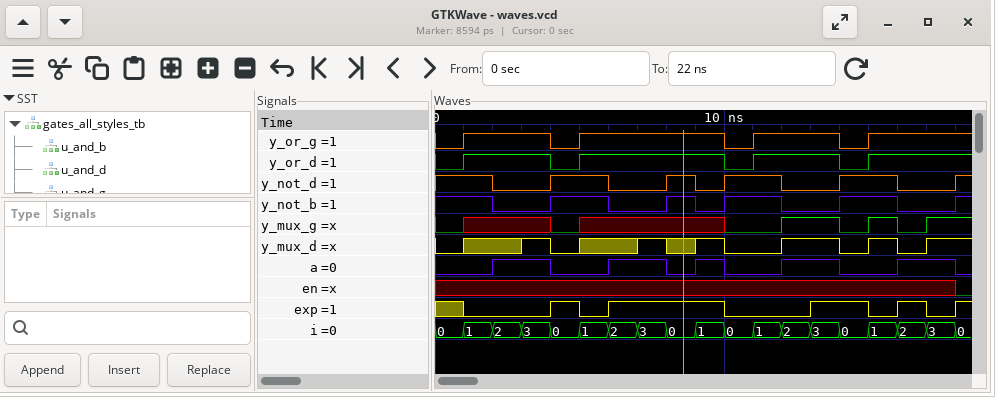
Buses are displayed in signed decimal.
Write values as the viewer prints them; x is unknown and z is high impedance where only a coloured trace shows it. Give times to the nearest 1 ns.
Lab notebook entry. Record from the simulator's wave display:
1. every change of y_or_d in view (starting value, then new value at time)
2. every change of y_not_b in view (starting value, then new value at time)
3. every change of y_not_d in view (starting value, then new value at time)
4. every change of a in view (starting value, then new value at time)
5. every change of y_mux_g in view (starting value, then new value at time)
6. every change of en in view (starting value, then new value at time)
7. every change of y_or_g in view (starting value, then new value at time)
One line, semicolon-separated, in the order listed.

0, 1 at 1 ns, 0 at 4 ns, 1 at 5 ns, 0 at 10 ns, 1 at 11 ns, 0 at 14 ns, 1 at 15 ns; 1, 0 at 2 ns, 1 at 4 ns, 0 at 6 ns, 1 at 8 ns, 0 at 9 ns, 1 at 10 ns, 0 at 12 ns, 1 at 14 ns, 0 at 16 ns, 1 at 18 ns; 1, 0 at 2 ns, 1 at 4 ns, 0 at 6 ns, 1 at 8 ns, 0 at 9 ns, 1 at 10 ns, 0 at 12 ns, 1 at 14 ns, 0 at 16 ns, 1 at 18 ns; 0, 1 at 2 ns, 0 at 4 ns, 1 at 6 ns, 0 at 8 ns, 1 at 9 ns, 0 at 10 ns, 1 at 12 ns, 0 at 14 ns, 1 at 16 ns, 0 at 18 ns; 0, x at 1 ns, 0 at 4 ns, x at 5 ns, 0 at 10 ns, 1 at 12 ns, 0 at 14 ns, 1 at 15 ns, 0 at 16 ns, 1 at 17 ns; x, 0 at 18 ns; 0, 1 at 1 ns, 0 at 4 ns, 1 at 5 ns, 0 at 10 ns, 1 at 11 ns, 0 at 14 ns, 1 at 15 ns
